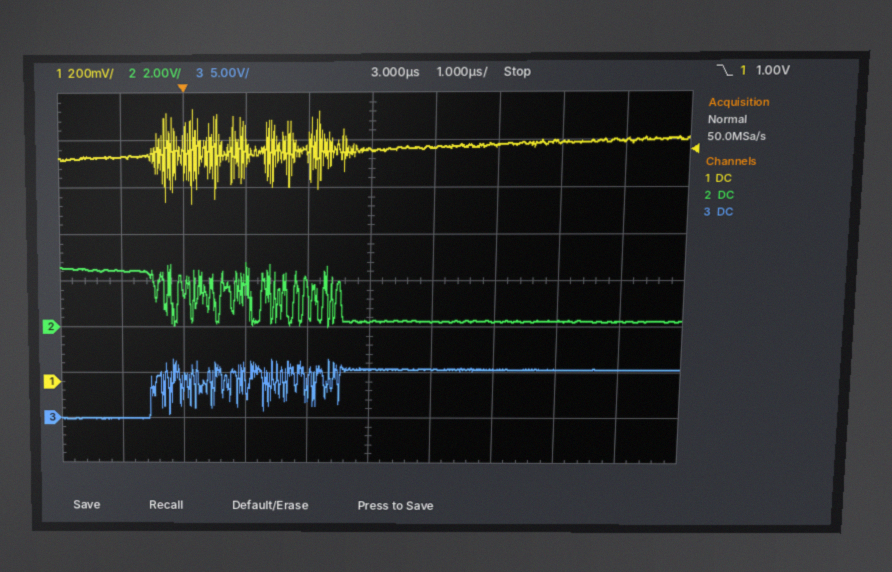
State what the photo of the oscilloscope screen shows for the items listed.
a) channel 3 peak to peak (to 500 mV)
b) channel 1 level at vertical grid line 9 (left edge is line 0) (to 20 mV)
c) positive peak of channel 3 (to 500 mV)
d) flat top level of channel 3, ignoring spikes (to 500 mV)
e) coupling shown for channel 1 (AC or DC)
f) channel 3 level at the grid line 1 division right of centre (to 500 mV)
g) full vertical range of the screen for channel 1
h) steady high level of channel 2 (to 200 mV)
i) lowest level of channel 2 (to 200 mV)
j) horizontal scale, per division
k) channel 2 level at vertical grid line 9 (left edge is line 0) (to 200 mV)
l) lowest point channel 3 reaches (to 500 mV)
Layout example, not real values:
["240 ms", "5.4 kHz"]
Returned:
["6.5 V", "1.04 V", "6.5 V", "5.5 V", "DC", "5.5 V", "1.6 V", "2.4 V", "0.0 V", "1 µs", "200 mV", "0.0 V"]
